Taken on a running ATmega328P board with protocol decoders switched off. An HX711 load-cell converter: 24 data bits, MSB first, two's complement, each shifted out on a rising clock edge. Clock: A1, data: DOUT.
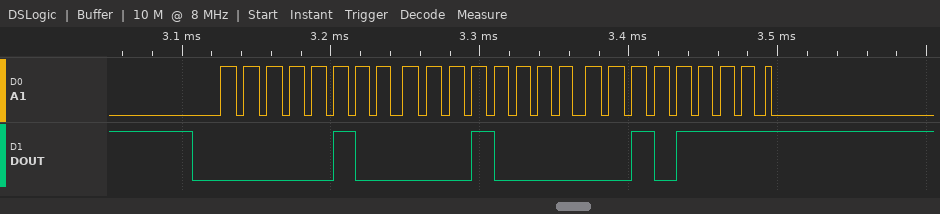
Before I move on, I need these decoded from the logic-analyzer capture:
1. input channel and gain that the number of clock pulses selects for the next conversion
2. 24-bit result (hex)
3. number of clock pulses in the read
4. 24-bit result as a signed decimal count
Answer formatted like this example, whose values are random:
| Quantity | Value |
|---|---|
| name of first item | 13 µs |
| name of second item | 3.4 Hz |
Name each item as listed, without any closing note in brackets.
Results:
| Quantity | Value |
|---|---|
| input channel and gain that the number of clock pulses selects for the next conversion | channel A, gain 128 |
| 24-bit result | 0x04102F |
| number of clock pulses in the read | 25 |
| 24-bit result as a signed decimal count | 266287 |
